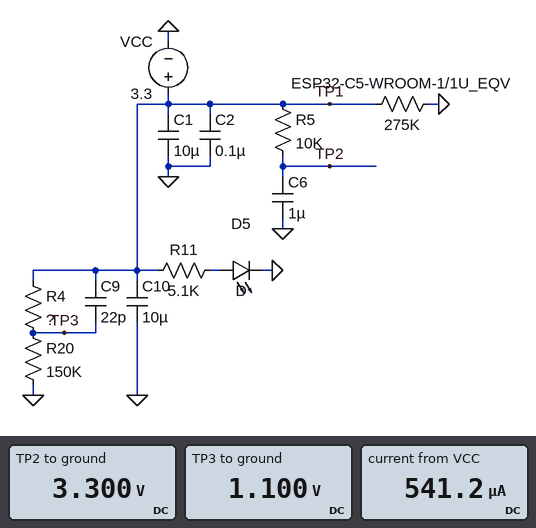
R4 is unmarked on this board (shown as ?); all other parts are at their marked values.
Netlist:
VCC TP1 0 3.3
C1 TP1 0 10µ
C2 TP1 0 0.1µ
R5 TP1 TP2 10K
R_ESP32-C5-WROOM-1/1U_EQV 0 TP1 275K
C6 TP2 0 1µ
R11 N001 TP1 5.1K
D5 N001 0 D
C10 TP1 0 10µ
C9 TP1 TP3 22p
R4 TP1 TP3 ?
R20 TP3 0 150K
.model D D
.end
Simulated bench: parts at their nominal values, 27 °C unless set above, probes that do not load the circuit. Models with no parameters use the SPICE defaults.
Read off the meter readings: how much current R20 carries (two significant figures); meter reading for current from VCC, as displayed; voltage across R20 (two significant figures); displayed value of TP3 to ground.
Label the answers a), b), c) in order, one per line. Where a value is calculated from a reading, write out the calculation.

a) (1.1 V) / 150 kΩ = 7.3 µA
b) 541.2 µA
c) 1.1 V = 1.1 V
d) 1.100 V
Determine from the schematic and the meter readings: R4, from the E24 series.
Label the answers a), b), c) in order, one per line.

a) 300 kΩ
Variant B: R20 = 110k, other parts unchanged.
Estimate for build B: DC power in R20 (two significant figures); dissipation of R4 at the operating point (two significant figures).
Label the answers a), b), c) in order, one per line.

a) 7.1 µW
b) 19 µW
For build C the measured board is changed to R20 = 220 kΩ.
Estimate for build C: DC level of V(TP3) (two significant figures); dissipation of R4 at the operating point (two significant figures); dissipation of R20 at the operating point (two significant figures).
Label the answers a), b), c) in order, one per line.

a) 1.4 V
b) 12 µW
c) 8.9 µW
